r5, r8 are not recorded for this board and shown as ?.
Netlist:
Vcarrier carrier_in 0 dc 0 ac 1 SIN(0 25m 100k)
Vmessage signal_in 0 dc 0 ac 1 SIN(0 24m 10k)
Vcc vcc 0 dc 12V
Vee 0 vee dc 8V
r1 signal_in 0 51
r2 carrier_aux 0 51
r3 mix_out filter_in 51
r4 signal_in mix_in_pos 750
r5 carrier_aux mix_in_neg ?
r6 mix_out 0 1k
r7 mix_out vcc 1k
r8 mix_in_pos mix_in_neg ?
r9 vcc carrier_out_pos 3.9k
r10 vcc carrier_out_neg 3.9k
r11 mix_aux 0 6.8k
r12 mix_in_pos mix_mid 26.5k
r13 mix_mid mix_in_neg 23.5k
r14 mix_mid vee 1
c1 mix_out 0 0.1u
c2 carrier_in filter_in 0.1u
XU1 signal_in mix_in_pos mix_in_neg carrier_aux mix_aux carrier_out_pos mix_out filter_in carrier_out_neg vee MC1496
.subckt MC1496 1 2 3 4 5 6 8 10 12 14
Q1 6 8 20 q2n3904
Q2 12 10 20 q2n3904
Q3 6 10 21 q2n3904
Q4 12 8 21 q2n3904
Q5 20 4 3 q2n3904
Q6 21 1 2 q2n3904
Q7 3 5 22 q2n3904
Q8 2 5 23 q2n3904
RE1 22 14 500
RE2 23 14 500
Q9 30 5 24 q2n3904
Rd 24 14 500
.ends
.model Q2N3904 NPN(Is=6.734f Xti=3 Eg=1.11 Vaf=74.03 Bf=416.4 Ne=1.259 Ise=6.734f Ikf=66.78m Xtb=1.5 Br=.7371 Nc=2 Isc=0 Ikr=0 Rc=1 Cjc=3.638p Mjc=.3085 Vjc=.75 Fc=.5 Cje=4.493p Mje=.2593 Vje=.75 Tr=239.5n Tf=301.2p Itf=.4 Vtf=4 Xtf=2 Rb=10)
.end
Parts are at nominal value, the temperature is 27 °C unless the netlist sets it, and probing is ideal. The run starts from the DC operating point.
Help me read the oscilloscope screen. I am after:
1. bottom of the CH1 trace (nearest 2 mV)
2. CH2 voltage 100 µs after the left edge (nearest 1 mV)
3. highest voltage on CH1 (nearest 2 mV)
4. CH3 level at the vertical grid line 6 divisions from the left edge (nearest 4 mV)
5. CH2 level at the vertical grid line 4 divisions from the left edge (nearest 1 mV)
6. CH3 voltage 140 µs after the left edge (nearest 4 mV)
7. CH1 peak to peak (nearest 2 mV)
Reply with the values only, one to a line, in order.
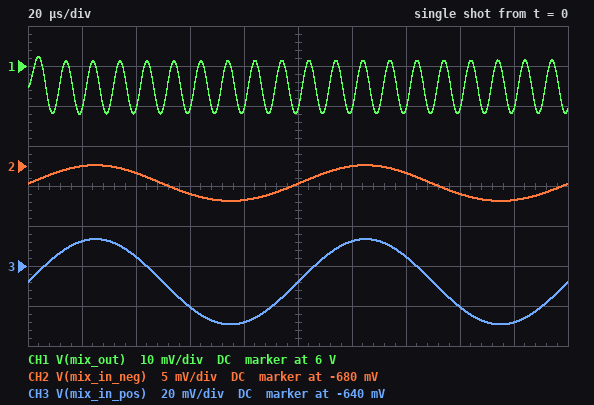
5.988 V
-682 mV
6.002 V
-628 mV
-684 mV
-636 mV
14 mV
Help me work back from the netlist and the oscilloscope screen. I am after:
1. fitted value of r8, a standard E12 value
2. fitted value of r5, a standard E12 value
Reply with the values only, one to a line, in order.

330 Ω
1.2 kΩ
